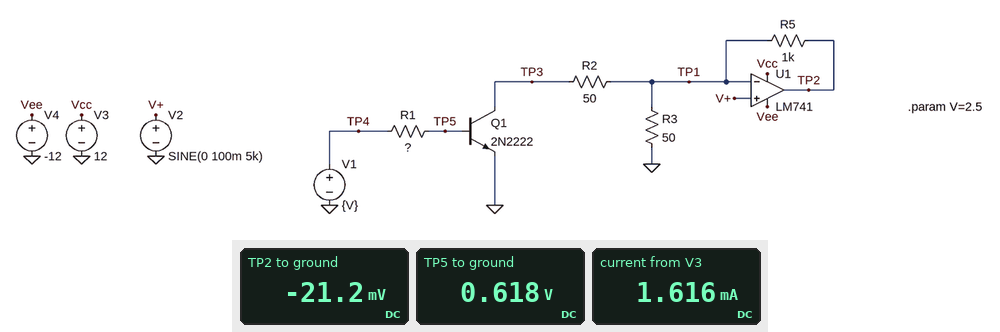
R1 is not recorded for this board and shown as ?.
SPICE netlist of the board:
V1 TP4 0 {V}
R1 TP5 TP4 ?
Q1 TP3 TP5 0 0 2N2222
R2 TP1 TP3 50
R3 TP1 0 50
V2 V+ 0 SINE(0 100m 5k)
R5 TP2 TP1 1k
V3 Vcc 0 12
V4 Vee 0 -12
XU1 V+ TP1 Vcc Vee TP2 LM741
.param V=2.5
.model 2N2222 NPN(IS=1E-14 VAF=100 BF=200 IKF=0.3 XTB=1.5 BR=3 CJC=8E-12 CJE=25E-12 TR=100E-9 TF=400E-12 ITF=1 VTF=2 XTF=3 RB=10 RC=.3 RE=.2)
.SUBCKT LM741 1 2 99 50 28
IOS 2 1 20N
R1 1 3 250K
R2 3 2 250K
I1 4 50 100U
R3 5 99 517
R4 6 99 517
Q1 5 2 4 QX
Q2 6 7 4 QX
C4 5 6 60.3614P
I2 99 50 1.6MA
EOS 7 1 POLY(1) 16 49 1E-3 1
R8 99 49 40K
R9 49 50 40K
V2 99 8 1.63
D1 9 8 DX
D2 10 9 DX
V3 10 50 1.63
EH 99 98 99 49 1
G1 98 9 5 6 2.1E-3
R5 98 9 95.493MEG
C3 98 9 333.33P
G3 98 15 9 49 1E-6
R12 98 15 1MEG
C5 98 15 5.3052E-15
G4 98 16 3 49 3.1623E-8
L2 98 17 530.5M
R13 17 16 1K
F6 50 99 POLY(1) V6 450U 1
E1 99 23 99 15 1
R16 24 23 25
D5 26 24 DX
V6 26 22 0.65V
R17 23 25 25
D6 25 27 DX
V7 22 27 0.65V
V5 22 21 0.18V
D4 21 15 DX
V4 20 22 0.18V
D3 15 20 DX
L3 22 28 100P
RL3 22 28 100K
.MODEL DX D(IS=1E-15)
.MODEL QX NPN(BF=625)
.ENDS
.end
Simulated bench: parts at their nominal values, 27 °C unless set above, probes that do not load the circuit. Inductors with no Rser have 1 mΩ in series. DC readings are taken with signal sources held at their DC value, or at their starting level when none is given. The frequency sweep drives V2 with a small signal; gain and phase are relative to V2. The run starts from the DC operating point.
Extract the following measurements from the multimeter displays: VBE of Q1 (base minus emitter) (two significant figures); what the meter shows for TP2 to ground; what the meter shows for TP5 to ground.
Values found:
620 mV
-21.2 mV
0.618 V
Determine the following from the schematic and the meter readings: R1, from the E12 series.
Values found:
27 kΩ
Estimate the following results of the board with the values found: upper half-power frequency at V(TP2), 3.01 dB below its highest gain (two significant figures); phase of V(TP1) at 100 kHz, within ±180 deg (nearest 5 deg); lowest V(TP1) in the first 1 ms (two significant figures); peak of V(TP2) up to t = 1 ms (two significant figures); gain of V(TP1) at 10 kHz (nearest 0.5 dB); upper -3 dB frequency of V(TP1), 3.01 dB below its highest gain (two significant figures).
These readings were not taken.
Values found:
32 kHz
-75 deg
-98 mV
3.1 V
-0.5 dB
32 kHz
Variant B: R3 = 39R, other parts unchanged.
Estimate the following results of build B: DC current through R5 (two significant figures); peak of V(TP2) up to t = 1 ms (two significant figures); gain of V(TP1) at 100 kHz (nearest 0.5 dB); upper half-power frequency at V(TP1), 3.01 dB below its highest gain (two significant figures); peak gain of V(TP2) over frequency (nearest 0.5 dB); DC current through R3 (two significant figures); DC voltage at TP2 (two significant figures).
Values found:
17 µA
3.6 V
-12.0 dB
26 kHz
30.5 dB
26 µA
-16 mV
